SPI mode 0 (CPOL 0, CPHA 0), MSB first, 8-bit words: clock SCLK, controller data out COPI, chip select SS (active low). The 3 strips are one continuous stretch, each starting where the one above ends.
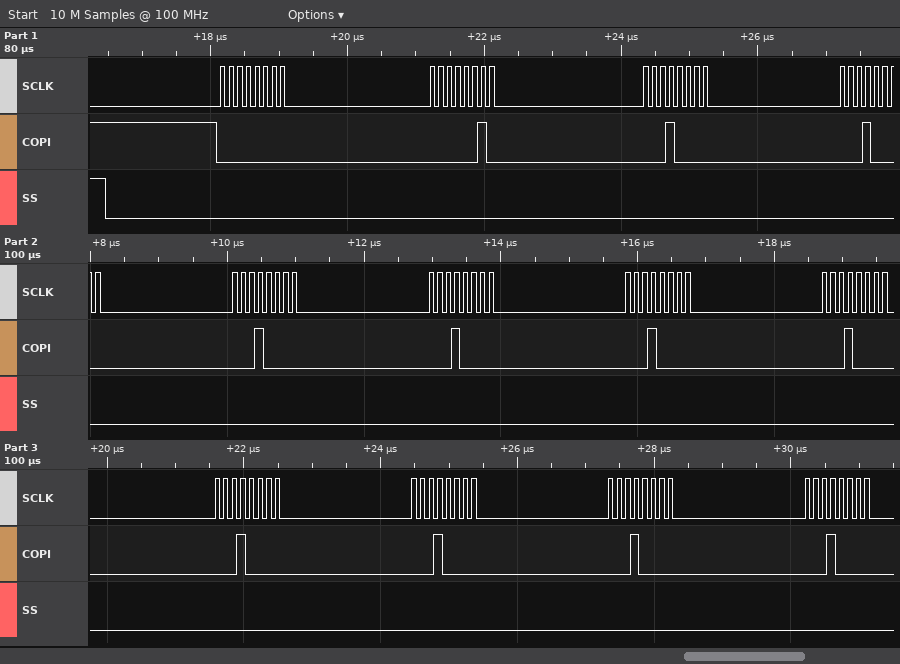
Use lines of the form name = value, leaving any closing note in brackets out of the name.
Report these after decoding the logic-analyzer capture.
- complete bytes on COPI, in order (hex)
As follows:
complete bytes on COPI, in order = 00 02 10 10 10 10 10 10 10 10 10 10
